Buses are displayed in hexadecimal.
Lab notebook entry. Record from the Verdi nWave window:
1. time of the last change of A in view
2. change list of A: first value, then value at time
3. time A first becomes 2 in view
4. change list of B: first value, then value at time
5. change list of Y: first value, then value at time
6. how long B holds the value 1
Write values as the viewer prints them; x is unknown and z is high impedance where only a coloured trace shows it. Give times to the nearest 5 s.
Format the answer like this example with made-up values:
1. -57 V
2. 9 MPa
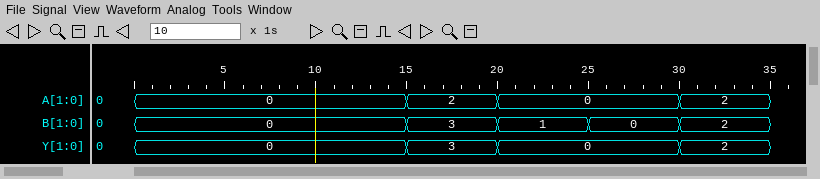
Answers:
1. 30 s
2. 0, 2 at 15 s, 0 at 20 s, 2 at 30 s
3. 15 s
4. 0, 3 at 15 s, 1 at 20 s, 0 at 25 s, 2 at 30 s
5. 0, 3 at 15 s, 0 at 20 s, 2 at 30 s
6. 5 s
